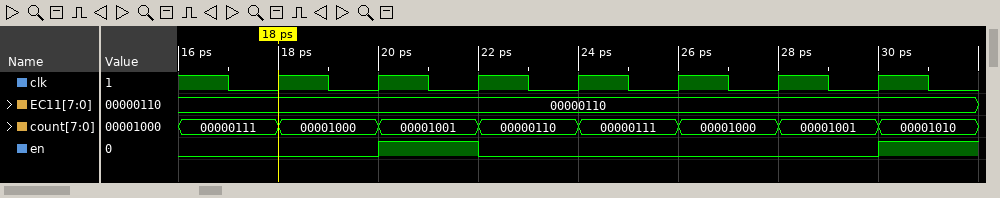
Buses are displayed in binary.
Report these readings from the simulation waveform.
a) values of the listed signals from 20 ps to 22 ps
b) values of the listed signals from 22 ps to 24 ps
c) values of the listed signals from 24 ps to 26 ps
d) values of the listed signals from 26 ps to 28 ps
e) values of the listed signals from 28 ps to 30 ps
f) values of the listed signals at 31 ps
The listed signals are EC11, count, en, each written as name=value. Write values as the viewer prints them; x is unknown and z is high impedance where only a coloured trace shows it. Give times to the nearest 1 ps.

EC11=00000110, count=00001001, en=1
EC11=00000110, count=00000110, en=0
EC11=00000110, count=00000111, en=0
EC11=00000110, count=00001000, en=0
EC11=00000110, count=00001001, en=0
EC11=00000110, count=00001010, en=1
